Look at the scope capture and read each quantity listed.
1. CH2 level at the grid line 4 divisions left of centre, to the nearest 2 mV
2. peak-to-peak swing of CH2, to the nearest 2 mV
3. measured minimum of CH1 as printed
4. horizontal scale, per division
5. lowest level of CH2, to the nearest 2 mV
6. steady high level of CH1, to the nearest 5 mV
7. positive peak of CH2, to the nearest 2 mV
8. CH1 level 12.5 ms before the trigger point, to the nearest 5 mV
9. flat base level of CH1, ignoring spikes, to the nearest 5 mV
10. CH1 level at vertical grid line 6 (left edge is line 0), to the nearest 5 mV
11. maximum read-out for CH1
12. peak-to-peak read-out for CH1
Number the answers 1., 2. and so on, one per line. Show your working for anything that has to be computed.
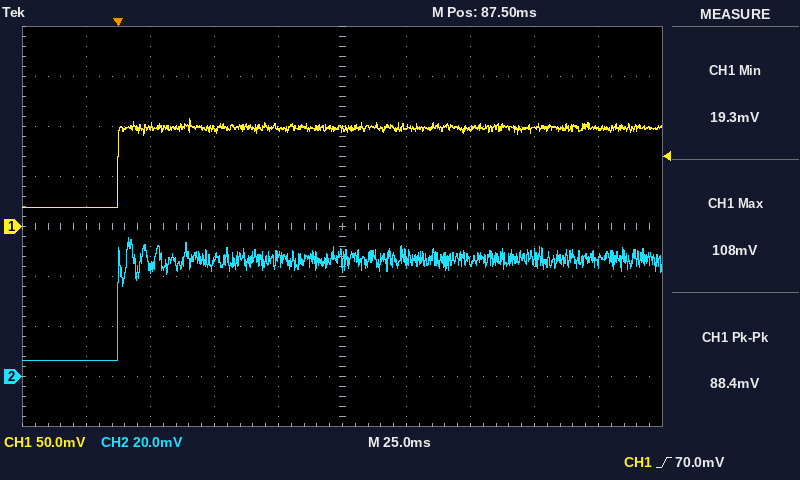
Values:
1. 6 mV
2. 56 mV − (6 mV) = 50 mV
3. 19.3 mV
4. 25 ms
5. 6 mV
6. 100 mV
7. 56 mV
8. 20 mV
9. 20 mV
10. 100 mV
11. 108 mV
12. 88.4 mV
